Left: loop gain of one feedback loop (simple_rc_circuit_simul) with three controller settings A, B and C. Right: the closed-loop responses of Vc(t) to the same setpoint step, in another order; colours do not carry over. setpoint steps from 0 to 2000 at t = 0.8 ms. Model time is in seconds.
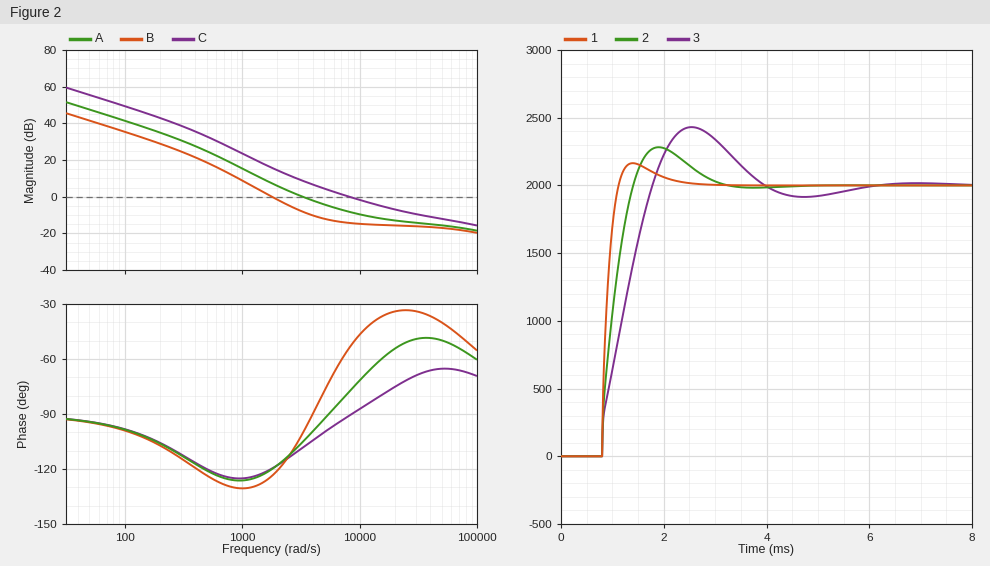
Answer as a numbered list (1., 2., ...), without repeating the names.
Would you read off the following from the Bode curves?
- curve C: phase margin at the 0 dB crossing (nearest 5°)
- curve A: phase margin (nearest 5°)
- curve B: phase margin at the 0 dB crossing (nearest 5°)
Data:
1. 90°
2. 75°
3. 55°
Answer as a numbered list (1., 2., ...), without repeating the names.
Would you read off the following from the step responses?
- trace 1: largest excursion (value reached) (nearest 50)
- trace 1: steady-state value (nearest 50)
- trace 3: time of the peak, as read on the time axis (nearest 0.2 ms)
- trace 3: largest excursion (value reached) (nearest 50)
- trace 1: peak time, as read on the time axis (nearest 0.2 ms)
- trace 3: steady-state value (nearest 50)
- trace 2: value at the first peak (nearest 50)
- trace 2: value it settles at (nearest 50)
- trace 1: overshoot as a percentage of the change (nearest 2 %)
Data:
1. 2150
2. 2000
3. 2.6 ms
4. 2450
5. 1.4 ms
6. 2000
7. 2300
8. 2000
9. 8 %
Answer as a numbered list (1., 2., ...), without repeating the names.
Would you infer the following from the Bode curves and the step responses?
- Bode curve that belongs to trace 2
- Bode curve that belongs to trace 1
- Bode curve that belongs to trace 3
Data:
1. A
2. C
3. B
